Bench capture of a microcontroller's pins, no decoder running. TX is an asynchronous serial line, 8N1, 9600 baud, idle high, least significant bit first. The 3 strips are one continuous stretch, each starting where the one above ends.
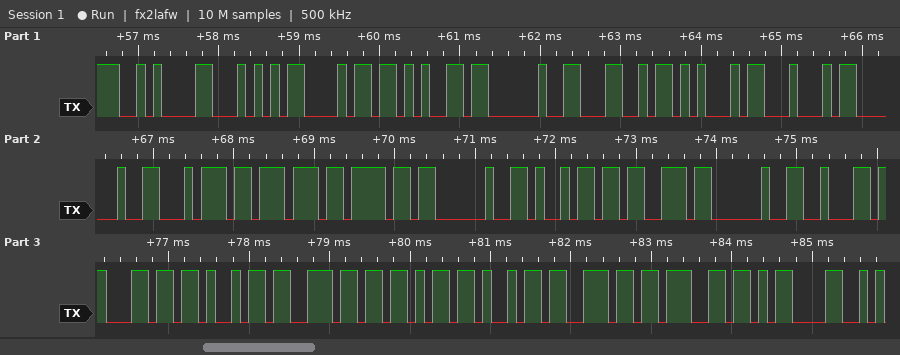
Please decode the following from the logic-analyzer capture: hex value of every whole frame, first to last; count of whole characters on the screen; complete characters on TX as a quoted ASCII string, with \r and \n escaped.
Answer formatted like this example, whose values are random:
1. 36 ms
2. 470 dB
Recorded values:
1. 0A 54 68 65 20 4C 45 44 20 74 77 6F 20 69 73 20 62 6C 69 6E 6B 69 6E 67 0D
2. 25
3. "\nThe LED two is blinking\r"
